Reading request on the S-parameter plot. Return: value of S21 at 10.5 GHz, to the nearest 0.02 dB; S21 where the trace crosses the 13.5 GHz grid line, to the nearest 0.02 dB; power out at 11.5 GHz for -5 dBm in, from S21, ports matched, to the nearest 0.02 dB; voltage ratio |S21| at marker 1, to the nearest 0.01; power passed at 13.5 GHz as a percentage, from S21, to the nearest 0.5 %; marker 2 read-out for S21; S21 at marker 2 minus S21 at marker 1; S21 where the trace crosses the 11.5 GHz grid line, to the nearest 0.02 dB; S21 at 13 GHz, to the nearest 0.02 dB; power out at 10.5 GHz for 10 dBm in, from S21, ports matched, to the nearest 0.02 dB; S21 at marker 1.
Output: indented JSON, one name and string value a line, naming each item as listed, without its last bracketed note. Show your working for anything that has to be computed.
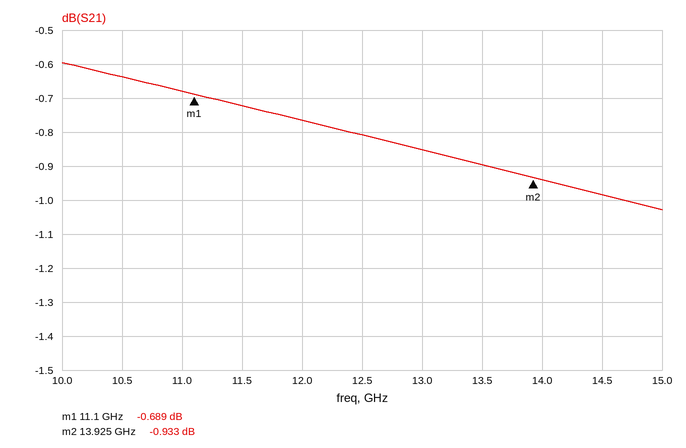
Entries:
{
  "value of S21 at 10.5 GHz, to the nearest 0.02 dB": "-0.64 dB",
  "S21 where the trace crosses the 13.5 GHz grid line, to the nearest 0.02 dB": "-0.90 dB",
  "power out at 11.5 GHz for -5 dBm in, from S21, ports matched, to the nearest 0.02 dB": "-5 dBm + (-0.72 dB) = -5.72 dBm",
  "voltage ratio |S21| at marker 1, to the nearest 0.01": "10^(-0.689/20) ≈ 0.92",
  "power passed at 13.5 GHz as a percentage, from S21, to the nearest 0.5 %": "10^(-0.9/10) ≈ 81.3 %, so 81.5 % to the nearest 0.5 %",
  "marker 2 read-out for S21": "-0.933 dB",
  "S21 at marker 2 minus S21 at marker 1": "-0.933 − (-0.689) = -0.244 dB",
  "S21 where the trace crosses the 11.5 GHz grid line, to the nearest 0.02 dB": "-0.72 dB",
  "S21 at 13 GHz, to the nearest 0.02 dB": "-0.86 dB",
  "power out at 10.5 GHz for 10 dBm in, from S21, ports matched, to the nearest 0.02 dB": "10 dBm + (-0.64 dB) = 9.36 dBm",
  "S21 at marker 1": "-0.689 dB"
}
